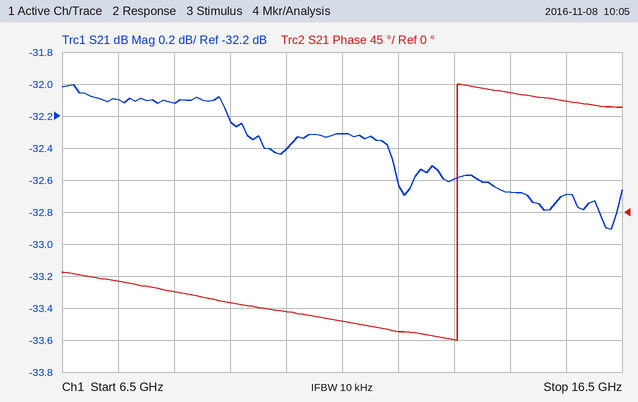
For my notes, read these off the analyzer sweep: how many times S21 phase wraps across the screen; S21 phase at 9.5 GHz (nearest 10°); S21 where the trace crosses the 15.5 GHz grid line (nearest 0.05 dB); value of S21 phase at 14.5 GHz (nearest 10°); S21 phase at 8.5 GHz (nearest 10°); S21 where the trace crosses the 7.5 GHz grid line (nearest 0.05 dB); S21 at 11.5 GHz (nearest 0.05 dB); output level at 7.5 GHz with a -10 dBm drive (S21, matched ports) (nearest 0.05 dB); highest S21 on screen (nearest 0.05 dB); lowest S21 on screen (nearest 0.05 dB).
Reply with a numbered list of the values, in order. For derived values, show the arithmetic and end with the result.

1. 1
2. -130°
3. -32.70 dB
4. 170°
5. -110°
6. -32.10 dB
7. -32.30 dB
8. -10 dBm + (-32.10 dB) = -42.10 dBm
9. -32.00 dB
10. -32.90 dB
